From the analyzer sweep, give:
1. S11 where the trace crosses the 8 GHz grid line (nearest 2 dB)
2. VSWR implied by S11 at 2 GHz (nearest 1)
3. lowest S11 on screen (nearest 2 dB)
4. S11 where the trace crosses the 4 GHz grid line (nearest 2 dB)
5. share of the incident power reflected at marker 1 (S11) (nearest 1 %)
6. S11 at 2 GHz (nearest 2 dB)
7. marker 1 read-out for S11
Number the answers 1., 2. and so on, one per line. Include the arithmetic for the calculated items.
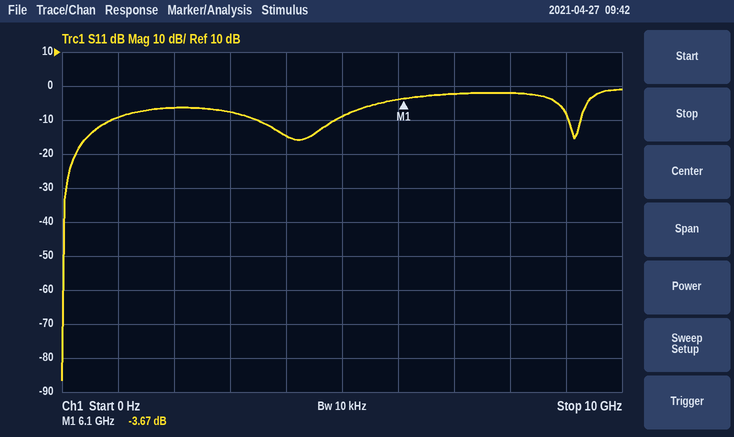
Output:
1. -2 dB
2. |Γ| = 10^(-6/20) = 0.5012; VSWR = (1 + 0.5012)/(1 − 0.5012) ≈ 3
3. -86 dB
4. -14 dB
5. 10^(-3.67/10) ≈ 43 %
6. -6 dB
7. -3.67 dB
